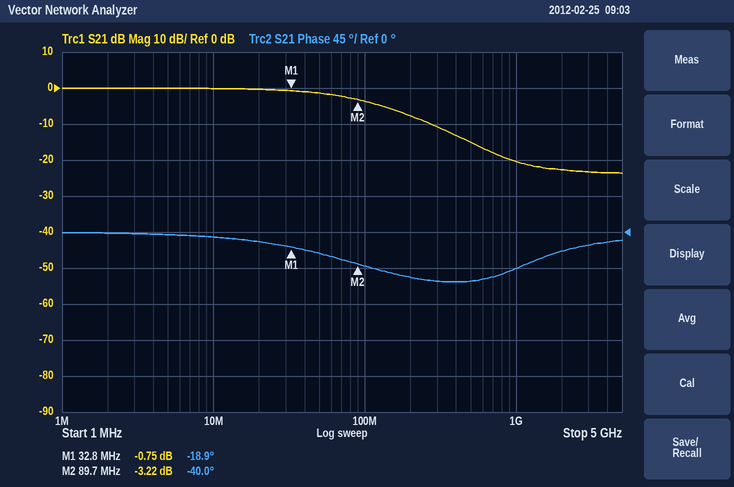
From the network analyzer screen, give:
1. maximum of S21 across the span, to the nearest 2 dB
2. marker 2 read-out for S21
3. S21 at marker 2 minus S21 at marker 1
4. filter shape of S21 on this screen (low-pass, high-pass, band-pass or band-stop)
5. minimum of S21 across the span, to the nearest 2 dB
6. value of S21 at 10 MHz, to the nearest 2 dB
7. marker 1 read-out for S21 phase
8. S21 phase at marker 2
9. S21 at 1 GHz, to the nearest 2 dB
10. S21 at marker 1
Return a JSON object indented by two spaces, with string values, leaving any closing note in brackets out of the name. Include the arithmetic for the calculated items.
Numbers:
{
  "maximum of S21 across the span, to the nearest 2 dB": "0 dB",
  "marker 2 read-out for S21": "-3.22 dB",
  "S21 at marker 2 minus S21 at marker 1": "-3.22 − (-0.75) = -2.47 dB",
  "filter shape of S21 on this screen": "low-pass",
  "minimum of S21 across the span, to the nearest 2 dB": "-24 dB",
  "value of S21 at 10 MHz, to the nearest 2 dB": "0 dB",
  "marker 1 read-out for S21 phase": "-18.9°",
  "S21 phase at marker 2": "-40.0°",
  "S21 at 1 GHz, to the nearest 2 dB": "-20 dB",
  "S21 at marker 1": "-0.75 dB"
}
